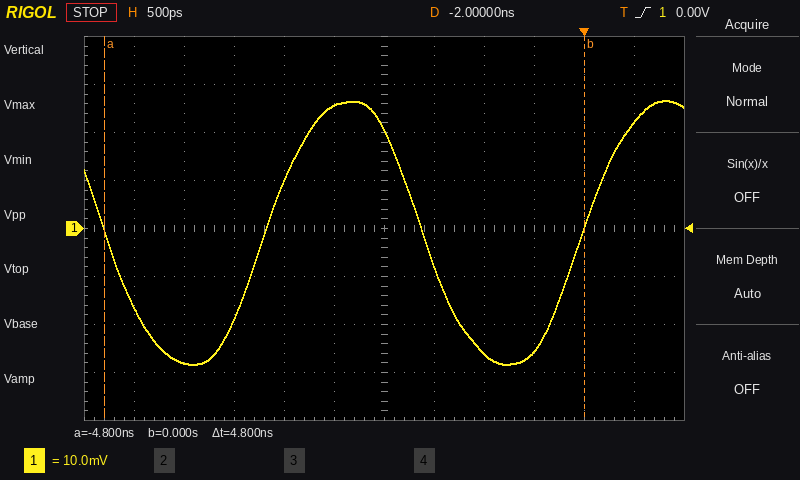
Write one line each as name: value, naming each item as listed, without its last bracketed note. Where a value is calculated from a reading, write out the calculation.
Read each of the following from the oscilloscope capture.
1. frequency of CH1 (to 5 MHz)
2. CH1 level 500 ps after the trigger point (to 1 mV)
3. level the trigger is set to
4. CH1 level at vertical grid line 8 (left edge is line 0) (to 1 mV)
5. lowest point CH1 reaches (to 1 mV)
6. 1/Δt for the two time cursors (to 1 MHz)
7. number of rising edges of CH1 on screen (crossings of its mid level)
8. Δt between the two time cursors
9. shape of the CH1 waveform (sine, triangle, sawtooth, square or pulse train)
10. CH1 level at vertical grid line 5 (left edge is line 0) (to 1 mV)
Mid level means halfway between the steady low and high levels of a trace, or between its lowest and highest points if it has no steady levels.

frequency of CH1: 315 MHz
CH1 level 500 ps after the trigger point: 22 mV
level the trigger is set to: 0.00 V
CH1 level at vertical grid line 8 (left edge is line 0): -26 mV
lowest point CH1 reaches: -28 mV
1/Δt for the two time cursors: 1 / 4.8 ns ≈ 208 MHz
number of rising edges of CH1 on screen: 2
Δt between the two time cursors: 4.8 ns
shape of the CH1 waveform: sine
CH1 level at vertical grid line 5 (left edge is line 0): 26 mV
